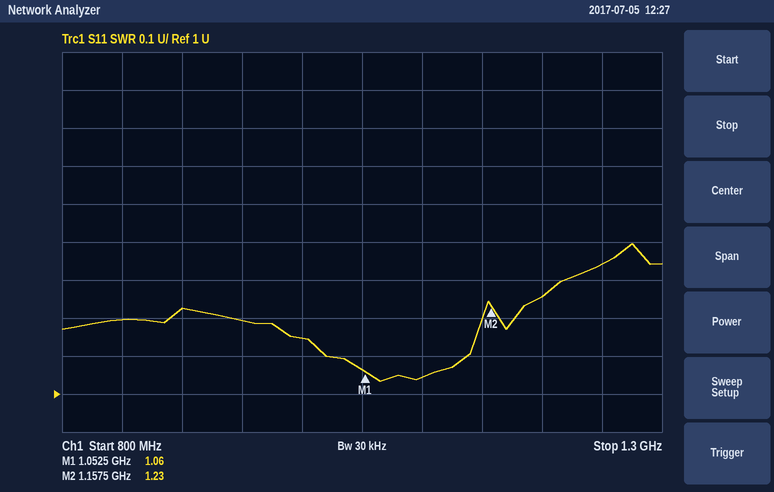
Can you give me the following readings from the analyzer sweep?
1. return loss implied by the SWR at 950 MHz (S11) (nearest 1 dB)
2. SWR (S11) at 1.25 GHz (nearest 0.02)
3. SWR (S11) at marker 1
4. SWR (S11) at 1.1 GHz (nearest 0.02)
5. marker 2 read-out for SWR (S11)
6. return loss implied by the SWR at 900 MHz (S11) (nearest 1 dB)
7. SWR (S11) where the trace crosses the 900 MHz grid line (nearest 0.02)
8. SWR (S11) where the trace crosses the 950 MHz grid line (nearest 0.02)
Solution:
21 dB
1.34
1.06
1.04
1.23
20 dB
1.22
1.20
